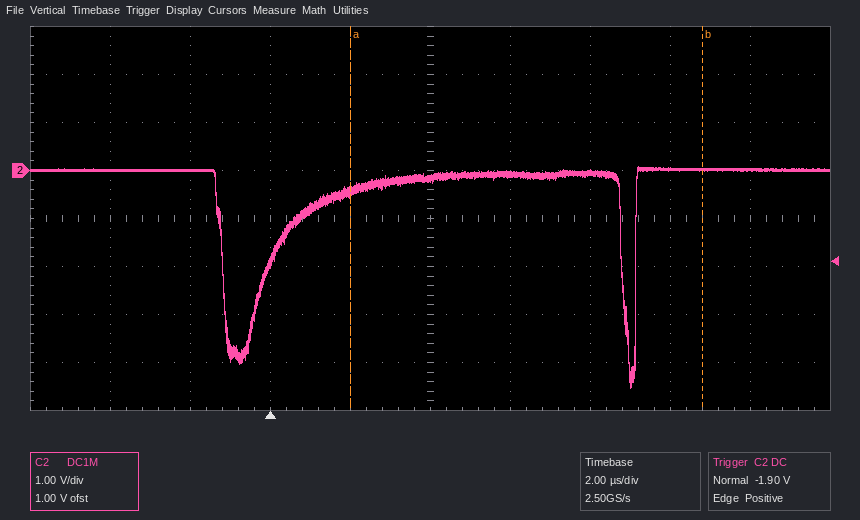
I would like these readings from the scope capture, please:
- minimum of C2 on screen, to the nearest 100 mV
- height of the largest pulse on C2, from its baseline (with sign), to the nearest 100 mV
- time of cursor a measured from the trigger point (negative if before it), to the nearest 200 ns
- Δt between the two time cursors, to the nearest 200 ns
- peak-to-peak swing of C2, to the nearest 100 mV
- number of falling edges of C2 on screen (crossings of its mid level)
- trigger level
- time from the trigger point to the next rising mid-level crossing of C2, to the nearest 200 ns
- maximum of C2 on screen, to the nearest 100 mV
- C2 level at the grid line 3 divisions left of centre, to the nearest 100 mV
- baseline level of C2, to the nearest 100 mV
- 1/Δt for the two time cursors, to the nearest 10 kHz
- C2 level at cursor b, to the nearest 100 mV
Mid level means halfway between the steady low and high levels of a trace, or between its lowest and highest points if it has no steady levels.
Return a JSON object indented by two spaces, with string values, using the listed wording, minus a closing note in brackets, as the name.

{
  "minimum of C2 on screen, to the nearest 100 mV": "-4.5 V",
  "height of the largest pulse on C2, from its baseline (with sign), to the nearest 100 mV": "-4.5 V",
  "time of cursor a measured from the trigger point (negative if before it), to the nearest 200 ns": "+2.0 µs",
  "Δt between the two time cursors, to the nearest 200 ns": "8.8 µs",
  "peak-to-peak swing of C2, to the nearest 100 mV": "4.6 V",
  "number of falling edges of C2 on screen": "2",
  "trigger level": "-1.90 V",
  "time from the trigger point to the next rising mid-level crossing of C2, to the nearest 200 ns": "9.2 µs",
  "maximum of C2 on screen, to the nearest 100 mV": "100 mV",
  "C2 level at the grid line 3 divisions left of centre, to the nearest 100 mV": "0.0 V",
  "baseline level of C2, to the nearest 100 mV": "0.0 V",
  "1/Δt for the two time cursors, to the nearest 10 kHz": "110 kHz",
  "C2 level at cursor b, to the nearest 100 mV": "0.0 V"
}
